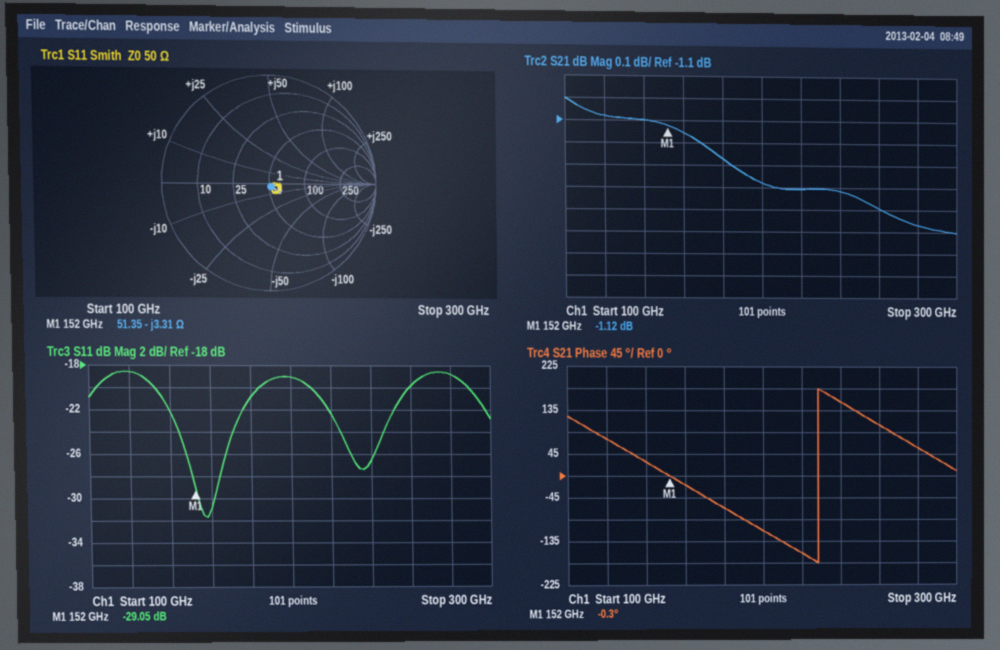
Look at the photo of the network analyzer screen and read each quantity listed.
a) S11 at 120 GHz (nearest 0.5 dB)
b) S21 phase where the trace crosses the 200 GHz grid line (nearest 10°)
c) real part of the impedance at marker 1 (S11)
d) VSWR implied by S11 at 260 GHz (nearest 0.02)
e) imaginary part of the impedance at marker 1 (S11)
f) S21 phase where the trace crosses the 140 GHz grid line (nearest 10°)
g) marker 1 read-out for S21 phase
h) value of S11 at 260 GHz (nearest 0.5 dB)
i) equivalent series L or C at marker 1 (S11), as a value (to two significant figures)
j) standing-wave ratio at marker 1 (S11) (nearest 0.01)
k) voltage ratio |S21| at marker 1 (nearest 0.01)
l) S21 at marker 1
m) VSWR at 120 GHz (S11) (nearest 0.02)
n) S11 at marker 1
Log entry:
-18.5 dB
-110°
51.35 Ω
1.22
-3.31 Ω
30°
-0.3°
-20.0 dB
320 fF
1.07
0.88
-1.12 dB
1.26
-29.05 dB
